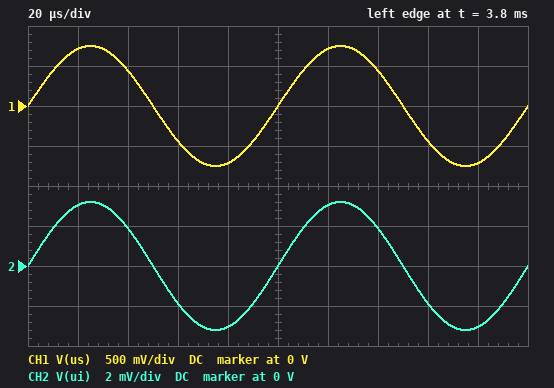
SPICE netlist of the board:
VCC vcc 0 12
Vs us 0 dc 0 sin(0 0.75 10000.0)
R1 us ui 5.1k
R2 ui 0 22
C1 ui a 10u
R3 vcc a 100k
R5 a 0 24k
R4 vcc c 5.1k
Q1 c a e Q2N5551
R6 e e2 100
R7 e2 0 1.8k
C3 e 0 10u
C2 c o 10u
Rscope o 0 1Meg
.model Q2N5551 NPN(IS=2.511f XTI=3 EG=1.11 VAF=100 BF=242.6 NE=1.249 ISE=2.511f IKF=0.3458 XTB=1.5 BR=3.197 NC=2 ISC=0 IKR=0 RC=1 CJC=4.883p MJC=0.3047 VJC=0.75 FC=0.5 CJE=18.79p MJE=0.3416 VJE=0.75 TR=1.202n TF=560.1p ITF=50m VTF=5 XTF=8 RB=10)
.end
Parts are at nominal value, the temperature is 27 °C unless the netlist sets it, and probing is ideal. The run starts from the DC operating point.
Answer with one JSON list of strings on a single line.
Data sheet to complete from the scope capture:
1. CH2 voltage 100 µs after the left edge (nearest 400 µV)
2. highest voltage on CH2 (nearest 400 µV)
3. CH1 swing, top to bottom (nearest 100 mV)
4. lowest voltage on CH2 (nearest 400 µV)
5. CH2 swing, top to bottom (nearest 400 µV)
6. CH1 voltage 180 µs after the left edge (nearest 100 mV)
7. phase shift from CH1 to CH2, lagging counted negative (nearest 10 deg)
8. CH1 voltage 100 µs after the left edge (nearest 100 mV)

["0 V", "3.2 mV", "1.5 V", "-3.2 mV", "6.4 mV", "-700 mV", "0 deg", "0 V"]
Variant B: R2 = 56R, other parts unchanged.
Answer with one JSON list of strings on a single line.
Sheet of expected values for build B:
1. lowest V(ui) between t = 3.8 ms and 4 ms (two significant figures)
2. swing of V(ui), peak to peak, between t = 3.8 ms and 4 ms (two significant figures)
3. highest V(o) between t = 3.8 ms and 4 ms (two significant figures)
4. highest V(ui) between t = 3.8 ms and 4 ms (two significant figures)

["-8.0 mV", "16 mV", "1.1 V", "8.0 mV"]
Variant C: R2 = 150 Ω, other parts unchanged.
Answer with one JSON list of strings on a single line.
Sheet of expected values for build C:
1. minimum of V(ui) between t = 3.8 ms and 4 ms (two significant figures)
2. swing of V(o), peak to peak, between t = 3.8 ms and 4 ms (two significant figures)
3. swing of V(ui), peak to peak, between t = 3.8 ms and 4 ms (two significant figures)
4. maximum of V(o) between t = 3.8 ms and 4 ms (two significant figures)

["-21 mV", "5.8 V", "41 mV", "2.4 V"]
